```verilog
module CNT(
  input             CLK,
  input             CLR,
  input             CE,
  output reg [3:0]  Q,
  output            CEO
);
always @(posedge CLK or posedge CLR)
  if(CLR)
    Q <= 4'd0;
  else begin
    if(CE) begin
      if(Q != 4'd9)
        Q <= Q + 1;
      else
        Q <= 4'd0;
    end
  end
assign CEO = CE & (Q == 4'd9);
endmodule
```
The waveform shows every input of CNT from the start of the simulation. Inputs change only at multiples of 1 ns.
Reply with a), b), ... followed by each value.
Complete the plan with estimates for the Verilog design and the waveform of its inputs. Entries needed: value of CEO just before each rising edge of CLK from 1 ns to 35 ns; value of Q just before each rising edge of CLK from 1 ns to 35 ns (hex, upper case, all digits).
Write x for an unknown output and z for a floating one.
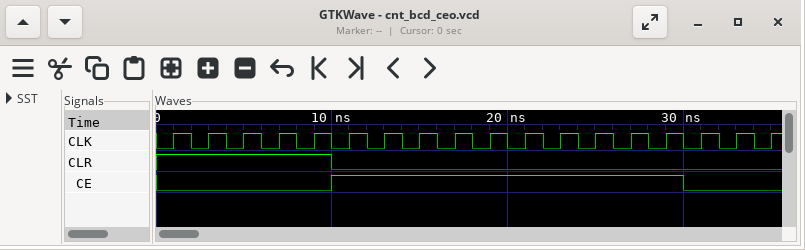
a) 0 0 0 0 0 0 0 0 0 0 0 0 0 0 1 0 0 0
b) 0, 0, 0, 0, 0, 0, 1, 2, 3, 4, 5, 6, 7, 8, 9, 0, 0, 0
